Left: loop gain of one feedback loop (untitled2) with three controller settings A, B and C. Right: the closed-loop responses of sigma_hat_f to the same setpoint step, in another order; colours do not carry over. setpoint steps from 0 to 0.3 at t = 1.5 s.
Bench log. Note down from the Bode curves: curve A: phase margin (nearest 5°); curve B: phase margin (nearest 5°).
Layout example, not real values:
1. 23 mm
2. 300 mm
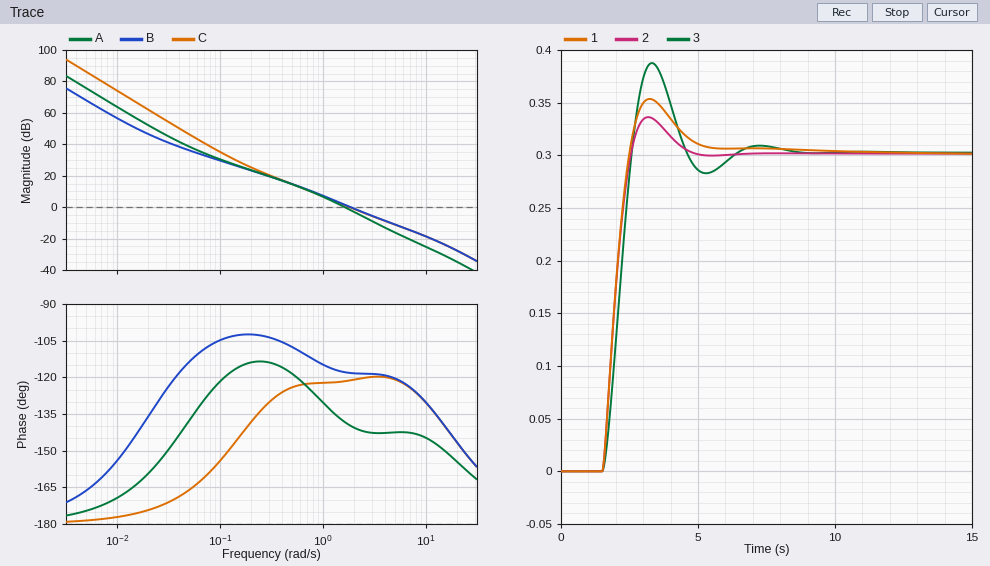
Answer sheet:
1. 40°
2. 60°
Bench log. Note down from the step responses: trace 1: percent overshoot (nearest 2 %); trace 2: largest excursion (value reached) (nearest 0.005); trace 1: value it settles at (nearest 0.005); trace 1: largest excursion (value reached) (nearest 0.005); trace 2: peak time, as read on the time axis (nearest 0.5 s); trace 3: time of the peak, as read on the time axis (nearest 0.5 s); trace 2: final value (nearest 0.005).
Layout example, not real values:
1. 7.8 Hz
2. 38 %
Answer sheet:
1. 18 %
2. 0.335
3. 0.300
4. 0.355
5. 3.0 s
6. 3.5 s
7. 0.300
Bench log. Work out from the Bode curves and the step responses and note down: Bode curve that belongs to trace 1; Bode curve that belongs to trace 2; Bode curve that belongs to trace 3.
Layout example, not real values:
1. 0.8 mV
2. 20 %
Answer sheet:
1. C
2. B
3. A
